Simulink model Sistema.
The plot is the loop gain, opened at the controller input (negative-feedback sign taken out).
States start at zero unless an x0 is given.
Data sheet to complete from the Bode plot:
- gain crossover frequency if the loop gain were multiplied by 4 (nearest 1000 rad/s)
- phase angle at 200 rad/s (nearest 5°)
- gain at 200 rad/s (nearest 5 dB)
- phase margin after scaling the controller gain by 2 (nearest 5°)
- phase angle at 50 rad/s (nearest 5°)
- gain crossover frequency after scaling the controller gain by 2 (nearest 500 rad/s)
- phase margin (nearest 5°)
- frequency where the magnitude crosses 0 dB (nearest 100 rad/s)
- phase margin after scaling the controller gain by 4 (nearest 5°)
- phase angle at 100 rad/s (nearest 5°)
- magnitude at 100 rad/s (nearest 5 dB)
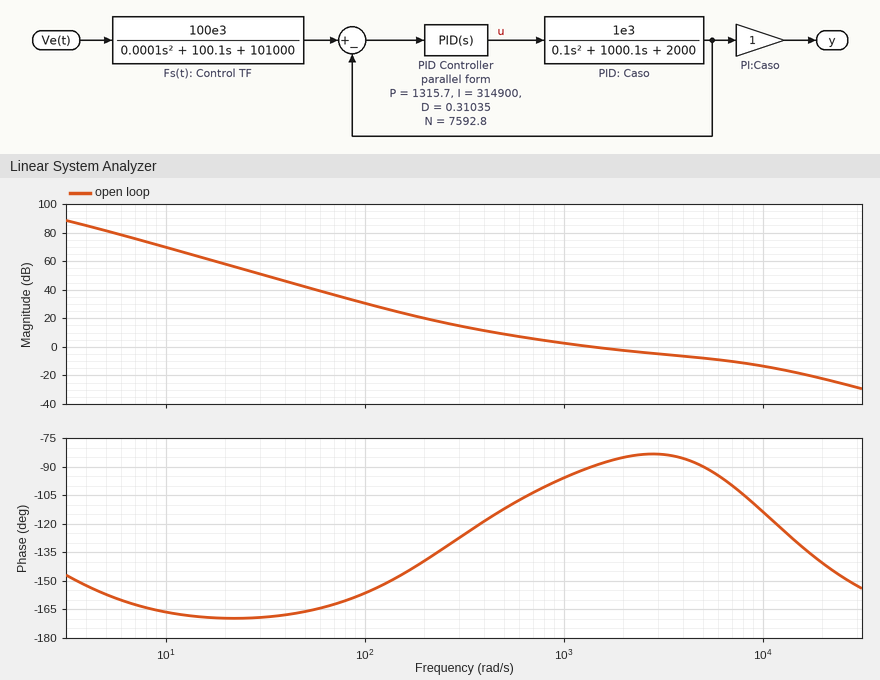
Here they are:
9000 rad/s
-140°
20 dB
95°
-165°
3500 rad/s
90°
1400 rad/s
70°
-155°
30 dB
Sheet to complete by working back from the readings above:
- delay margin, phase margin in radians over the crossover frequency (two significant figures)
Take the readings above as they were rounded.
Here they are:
0.0011 s
